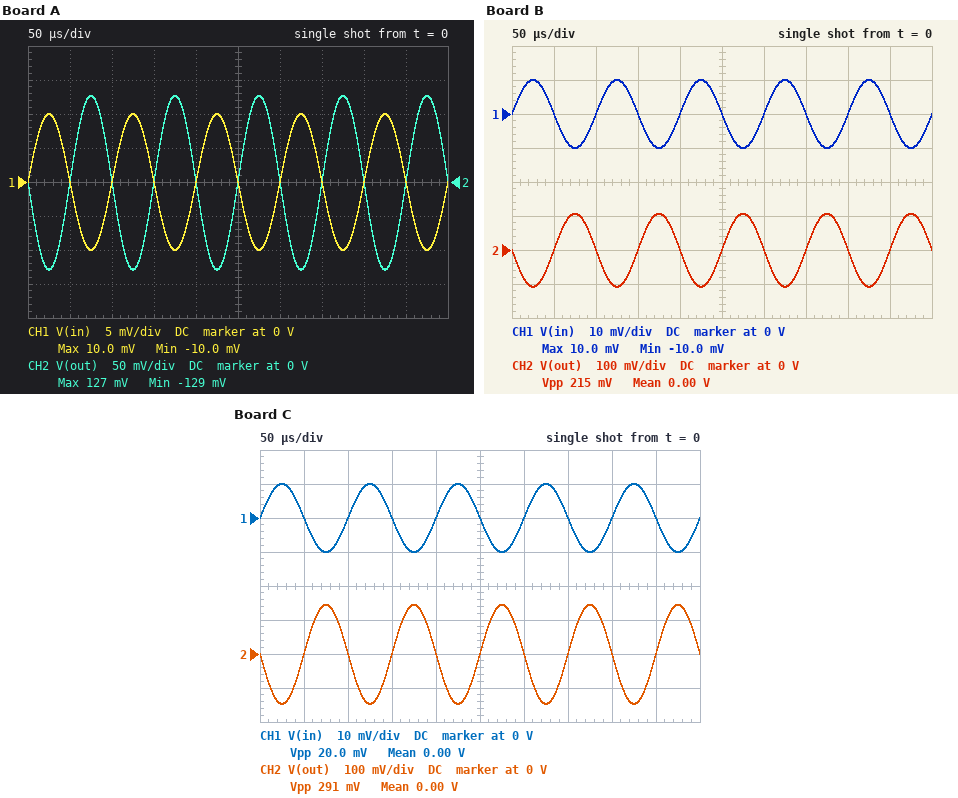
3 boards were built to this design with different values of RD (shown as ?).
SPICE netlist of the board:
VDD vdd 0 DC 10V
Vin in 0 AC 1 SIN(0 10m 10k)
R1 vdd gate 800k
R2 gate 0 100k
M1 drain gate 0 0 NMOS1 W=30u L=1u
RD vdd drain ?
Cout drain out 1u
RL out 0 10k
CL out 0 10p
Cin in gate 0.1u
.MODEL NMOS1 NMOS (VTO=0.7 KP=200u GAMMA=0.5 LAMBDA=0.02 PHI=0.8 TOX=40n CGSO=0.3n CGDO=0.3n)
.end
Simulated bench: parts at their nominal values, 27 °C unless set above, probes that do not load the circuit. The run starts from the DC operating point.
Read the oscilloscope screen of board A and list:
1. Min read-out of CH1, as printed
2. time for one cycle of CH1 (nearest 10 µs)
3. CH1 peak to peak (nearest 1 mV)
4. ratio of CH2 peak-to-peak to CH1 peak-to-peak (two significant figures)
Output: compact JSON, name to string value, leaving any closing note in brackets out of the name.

{"Min read-out of CH1, as printed": "-10.0 mV", "time for one cycle of CH1": "100 µs", "CH1 peak to peak": "20 mV", "ratio of CH2 peak-to-peak to CH1 peak-to-peak": "13"}
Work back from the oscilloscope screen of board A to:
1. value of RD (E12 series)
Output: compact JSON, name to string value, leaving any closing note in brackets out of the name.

{"value of RD": "10 kΩ"}
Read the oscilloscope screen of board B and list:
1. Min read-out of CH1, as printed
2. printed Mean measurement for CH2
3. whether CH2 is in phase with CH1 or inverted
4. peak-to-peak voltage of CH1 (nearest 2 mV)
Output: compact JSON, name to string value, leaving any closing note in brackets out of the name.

{"Min read-out of CH1, as printed": "-10.0 mV", "printed Mean measurement for CH2": "0.00 V", "whether CH2 is in phase with CH1 or inverted": "inverted", "peak-to-peak voltage of CH1": "20 mV"}
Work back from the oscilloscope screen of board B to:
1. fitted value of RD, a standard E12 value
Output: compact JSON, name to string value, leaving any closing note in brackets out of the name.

{"fitted value of RD, a standard E12 value": "6.8 kΩ"}
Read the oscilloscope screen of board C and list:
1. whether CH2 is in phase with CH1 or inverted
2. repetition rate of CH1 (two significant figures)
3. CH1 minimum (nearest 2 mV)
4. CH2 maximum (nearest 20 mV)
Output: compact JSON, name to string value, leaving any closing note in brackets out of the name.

{"whether CH2 is in phase with CH1 or inverted": "inverted", "repetition rate of CH1": "10 kHz", "CH1 minimum": "-10 mV", "CH2 maximum": "140 mV"}
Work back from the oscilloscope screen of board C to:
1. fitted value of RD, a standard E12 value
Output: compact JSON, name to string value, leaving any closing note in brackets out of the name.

{"fitted value of RD, a standard E12 value": "15 kΩ"}
